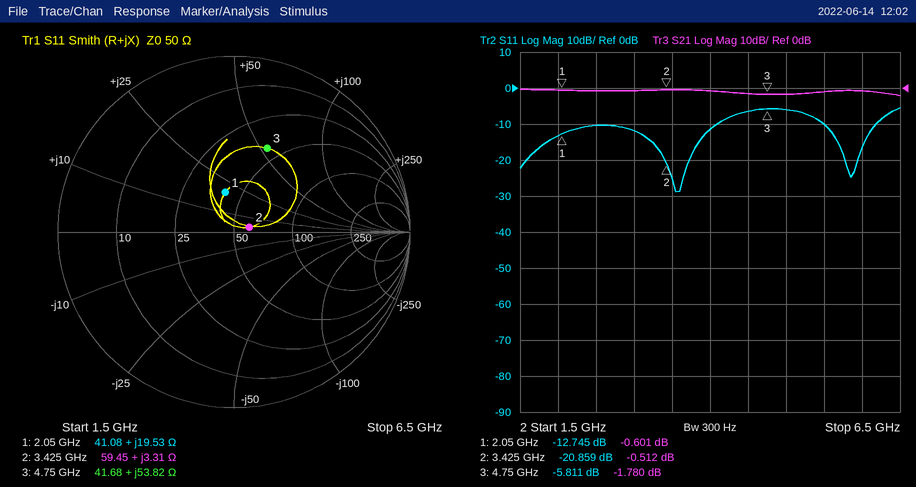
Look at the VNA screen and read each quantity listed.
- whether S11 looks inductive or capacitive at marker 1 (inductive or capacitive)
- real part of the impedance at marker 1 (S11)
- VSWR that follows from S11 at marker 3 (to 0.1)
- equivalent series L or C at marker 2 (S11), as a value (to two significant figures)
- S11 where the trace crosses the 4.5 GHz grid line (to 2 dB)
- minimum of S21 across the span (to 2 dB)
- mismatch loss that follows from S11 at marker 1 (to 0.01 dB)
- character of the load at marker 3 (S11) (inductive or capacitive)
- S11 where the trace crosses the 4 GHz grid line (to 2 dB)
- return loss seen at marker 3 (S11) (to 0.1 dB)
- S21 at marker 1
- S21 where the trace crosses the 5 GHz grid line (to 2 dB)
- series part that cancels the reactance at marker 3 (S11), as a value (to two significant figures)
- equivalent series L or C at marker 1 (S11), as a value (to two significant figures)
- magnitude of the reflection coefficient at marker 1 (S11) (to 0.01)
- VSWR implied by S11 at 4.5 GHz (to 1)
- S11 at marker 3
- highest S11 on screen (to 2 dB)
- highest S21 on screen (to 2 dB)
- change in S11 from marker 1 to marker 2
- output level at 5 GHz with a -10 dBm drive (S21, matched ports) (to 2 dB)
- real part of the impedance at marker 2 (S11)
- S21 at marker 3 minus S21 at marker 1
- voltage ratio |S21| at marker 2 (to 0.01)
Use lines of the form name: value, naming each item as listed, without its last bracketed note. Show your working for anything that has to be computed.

whether S11 looks inductive or capacitive at marker 1: inductive
real part of the impedance at marker 1: 41.08 Ω
VSWR that follows from S11 at marker 3: (1 + 0.5122)/(1 − 0.5122) ≈ 3.1
equivalent series L or C at marker 2 (S11), as a value: L = 3.31 Ω/(2π × 3.425 GHz) ≈ 154 pH, so 150 pH to two significant figures
S11 where the trace crosses the 4.5 GHz grid line: -6 dB
minimum of S21 across the span: -2 dB
mismatch loss that follows from S11 at marker 1: −10 log10(1 − 10^(-12.745/10)) ≈ 0.24 dB
character of the load at marker 3 (S11): inductive
S11 where the trace crosses the 4 GHz grid line: -12 dB
return loss seen at marker 3 (S11): 5.8 dB
S21 at marker 1: -0.601 dB
S21 where the trace crosses the 5 GHz grid line: -2 dB
series part that cancels the reactance at marker 3 (S11), as a value: C = 1/(2π × 4.75 GHz × 53.82 Ω) ≈ 623 fF, so 620 fF to two significant figures
equivalent series L or C at marker 1 (S11), as a value: L = 19.53 Ω/(2π × 2.05 GHz) ≈ 1.5 nH
magnitude of the reflection coefficient at marker 1 (S11): 0.23
VSWR implied by S11 at 4.5 GHz: |Γ| = 10^(-6/20) = 0.5012; VSWR = (1 + 0.5012)/(1 − 0.5012) ≈ 3
S11 at marker 3: -5.811 dB
highest S11 on screen: -6 dB
highest S21 on screen: 0 dB
change in S11 from marker 1 to marker 2: -20.859 − (-12.745) = -8.114 dB
output level at 5 GHz with a -10 dBm drive (S21, matched ports): -10 dBm + (-2 dB) = -12 dBm
real part of the impedance at marker 2: 59.45 Ω
S21 at marker 3 minus S21 at marker 1: -1.78 − (-0.601) = -1.179 dB
voltage ratio |S21| at marker 2: 10^(-0.512/20) ≈ 0.94
